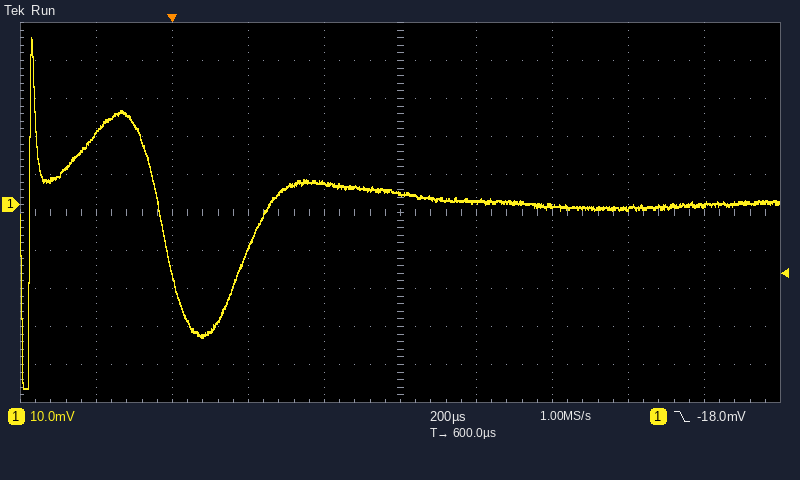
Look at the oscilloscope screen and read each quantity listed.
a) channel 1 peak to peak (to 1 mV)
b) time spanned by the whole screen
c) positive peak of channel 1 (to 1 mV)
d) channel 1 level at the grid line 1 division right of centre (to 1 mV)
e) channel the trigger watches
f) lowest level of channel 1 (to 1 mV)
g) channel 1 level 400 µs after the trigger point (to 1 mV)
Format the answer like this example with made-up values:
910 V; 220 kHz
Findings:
92 mV; 2 ms; 44 mV; 1 mV; channel 1; -48 mV; 6 mV
